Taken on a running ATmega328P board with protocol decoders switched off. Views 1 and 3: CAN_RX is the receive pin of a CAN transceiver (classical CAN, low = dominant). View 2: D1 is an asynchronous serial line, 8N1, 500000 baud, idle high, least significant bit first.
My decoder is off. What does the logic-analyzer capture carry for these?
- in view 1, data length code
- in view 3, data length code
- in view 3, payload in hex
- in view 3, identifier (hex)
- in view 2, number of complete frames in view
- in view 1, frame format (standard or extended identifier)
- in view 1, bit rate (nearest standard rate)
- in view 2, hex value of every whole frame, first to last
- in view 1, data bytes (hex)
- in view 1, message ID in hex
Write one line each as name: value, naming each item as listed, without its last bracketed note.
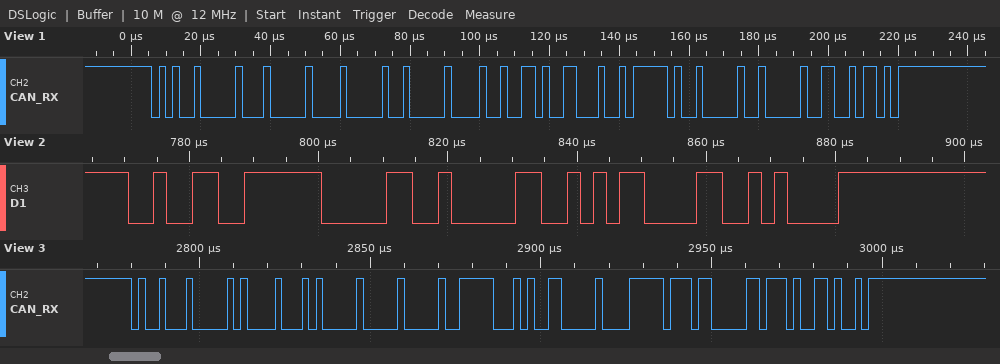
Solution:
in view 1, data length code: 8
in view 3, data length code: 8
in view 3, payload in hex: 45 00 00 7C A6 00 FF 60
in view 3, identifier: 0x488
in view 2, number of complete frames in view: 5
in view 1, frame format: standard
in view 1, bit rate: 500 kbit/s
in view 2, hex value of every whole frame, first to last: 32 30 30 0D 0A
in view 1, data bytes: 02 02 00 93 4C 4B F2 02
in view 1, message ID in hex: 0x520
